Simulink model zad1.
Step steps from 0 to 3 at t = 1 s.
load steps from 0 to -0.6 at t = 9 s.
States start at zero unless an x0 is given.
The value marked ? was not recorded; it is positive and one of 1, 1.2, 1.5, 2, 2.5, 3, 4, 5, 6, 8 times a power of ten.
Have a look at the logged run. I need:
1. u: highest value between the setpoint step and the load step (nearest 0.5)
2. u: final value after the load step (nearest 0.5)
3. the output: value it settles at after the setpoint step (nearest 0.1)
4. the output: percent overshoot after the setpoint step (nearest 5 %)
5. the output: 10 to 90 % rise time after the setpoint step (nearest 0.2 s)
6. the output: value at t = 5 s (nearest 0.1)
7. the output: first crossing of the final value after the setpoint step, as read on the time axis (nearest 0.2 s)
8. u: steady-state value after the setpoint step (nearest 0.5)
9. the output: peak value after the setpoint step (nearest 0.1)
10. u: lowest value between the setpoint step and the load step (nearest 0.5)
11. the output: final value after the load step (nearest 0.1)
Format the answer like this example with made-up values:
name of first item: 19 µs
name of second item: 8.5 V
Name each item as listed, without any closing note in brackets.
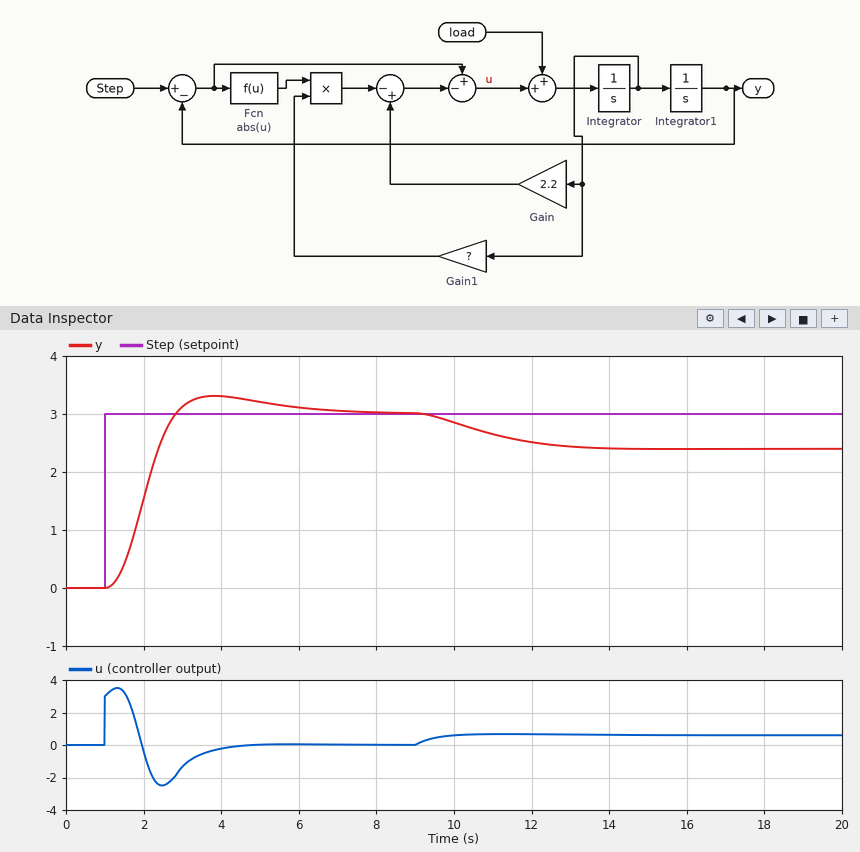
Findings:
u: highest value between the setpoint step and the load step: 3.5
u: final value after the load step: 0.5
the output: value it settles at after the setpoint step: 3.0
the output: percent overshoot after the setpoint step: 10 %
the output: 10 to 90 % rise time after the setpoint step: 1.2 s
the output: value at t = 5 s: 3.2
the output: first crossing of the final value after the setpoint step, as read on the time axis: 2.8 s
u: steady-state value after the setpoint step: 0.0
the output: peak value after the setpoint step: 3.3
u: lowest value between the setpoint step and the load step: -2.5
the output: final value after the load step: 2.4
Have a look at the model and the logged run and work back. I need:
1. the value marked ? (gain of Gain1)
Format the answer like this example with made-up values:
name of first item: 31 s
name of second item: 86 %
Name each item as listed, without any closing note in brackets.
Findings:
the value marked ?: 1
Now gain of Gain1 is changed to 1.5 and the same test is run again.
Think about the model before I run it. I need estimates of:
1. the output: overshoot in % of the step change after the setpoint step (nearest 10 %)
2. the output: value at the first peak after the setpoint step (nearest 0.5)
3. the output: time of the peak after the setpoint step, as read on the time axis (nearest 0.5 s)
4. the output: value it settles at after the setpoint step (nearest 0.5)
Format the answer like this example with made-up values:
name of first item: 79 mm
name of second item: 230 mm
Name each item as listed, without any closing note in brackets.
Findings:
the output: overshoot in % of the step change after the setpoint step: 40 %
the output: value at the first peak after the setpoint step: 4.0
the output: time of the peak after the setpoint step, as read on the time axis: 3.5 s
the output: value it settles at after the setpoint step: 3.0
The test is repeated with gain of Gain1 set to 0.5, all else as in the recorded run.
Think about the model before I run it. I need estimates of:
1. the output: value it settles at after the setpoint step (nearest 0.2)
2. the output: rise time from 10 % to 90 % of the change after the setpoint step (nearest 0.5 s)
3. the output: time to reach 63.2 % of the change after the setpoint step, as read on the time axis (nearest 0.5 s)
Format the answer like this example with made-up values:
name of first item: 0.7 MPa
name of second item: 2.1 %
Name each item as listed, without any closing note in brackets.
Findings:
the output: value it settles at after the setpoint step: 3.0
the output: rise time from 10 % to 90 % of the change after the setpoint step: 2.0 s
the output: time to reach 63.2 % of the change after the setpoint step, as read on the time axis: 2.5 s
